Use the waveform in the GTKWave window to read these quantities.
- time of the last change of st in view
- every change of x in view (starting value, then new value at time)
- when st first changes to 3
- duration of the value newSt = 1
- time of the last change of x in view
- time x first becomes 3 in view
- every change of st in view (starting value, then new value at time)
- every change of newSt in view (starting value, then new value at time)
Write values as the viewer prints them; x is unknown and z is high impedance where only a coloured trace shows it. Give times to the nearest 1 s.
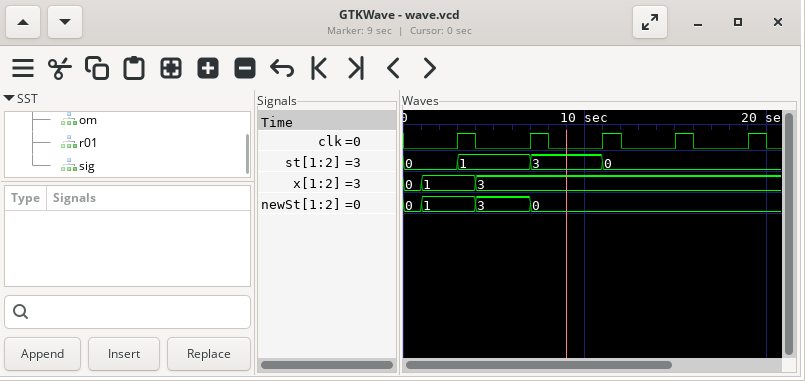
11 s
0, 1 at 1 s, 3 at 4 s
7 s
3 s
4 s
4 s
0, 1 at 3 s, 3 at 7 s, 0 at 11 s
0, 1 at 1 s, 3 at 4 s, 0 at 7 s
